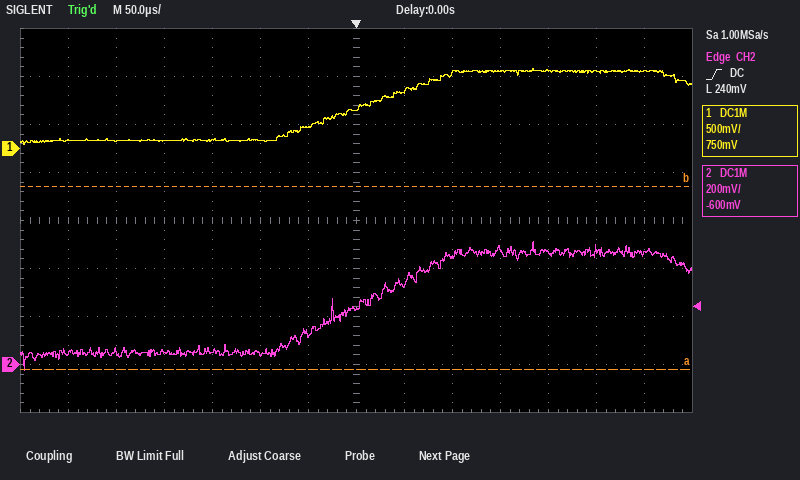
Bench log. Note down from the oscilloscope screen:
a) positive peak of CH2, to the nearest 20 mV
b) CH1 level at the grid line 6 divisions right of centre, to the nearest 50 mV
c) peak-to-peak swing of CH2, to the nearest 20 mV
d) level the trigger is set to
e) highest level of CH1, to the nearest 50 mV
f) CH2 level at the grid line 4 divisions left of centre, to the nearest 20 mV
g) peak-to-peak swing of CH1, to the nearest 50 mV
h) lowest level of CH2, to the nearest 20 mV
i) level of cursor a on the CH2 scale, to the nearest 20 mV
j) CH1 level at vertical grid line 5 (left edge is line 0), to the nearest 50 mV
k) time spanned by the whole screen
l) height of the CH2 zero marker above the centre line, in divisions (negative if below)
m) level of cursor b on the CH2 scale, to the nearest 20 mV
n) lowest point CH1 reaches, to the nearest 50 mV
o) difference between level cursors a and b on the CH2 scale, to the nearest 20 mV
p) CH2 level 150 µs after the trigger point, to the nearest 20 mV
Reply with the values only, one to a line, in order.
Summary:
520 mV
800 mV
540 mV
240 mV
850 mV
60 mV
800 mV
-20 mV
-20 mV
100 mV
700 µs
-3.0 div
740 mV
50 mV
760 mV
480 mV
